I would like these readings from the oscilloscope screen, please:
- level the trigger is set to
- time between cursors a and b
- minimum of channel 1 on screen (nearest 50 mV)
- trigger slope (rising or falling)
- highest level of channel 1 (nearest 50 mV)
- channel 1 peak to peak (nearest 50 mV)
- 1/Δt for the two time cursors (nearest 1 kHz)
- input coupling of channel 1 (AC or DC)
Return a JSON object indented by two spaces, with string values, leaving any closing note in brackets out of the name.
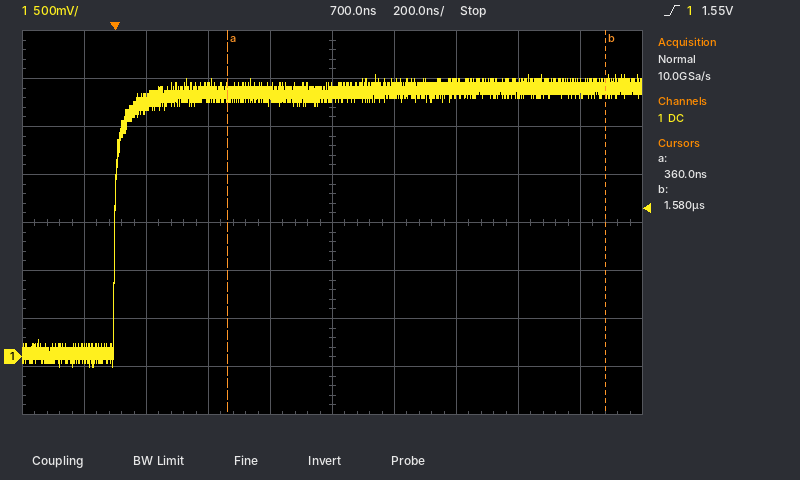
{
  "level the trigger is set to": "1.55 V",
  "time between cursors a and b": "1.22 µs",
  "minimum of channel 1 on screen": "-100 mV",
  "trigger slope": "rising",
  "highest level of channel 1": "2.95 V",
  "channel 1 peak to peak": "3.05 V",
  "1/Δt for the two time cursors": "820 kHz",
  "input coupling of channel 1": "DC"
}
